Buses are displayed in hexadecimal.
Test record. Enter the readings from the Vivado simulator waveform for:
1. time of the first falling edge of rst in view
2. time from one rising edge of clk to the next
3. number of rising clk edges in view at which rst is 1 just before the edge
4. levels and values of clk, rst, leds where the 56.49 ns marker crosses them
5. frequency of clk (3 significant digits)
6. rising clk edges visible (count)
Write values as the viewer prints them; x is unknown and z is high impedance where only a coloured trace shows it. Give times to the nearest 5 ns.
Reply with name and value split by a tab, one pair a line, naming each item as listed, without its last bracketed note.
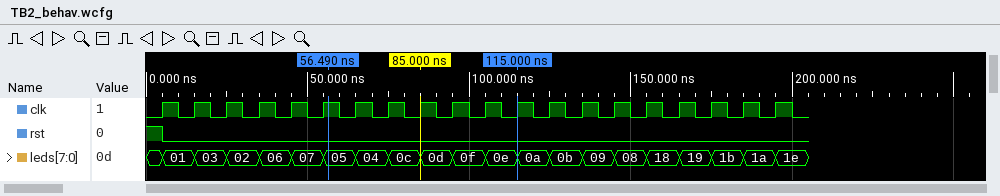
time of the first falling edge of rst in view	5 ns
time from one rising edge of clk to the next	10 ns
number of rising clk edges in view at which rst is 1 just before the edge	1
levels and values of clk, rst, leds where the 56.49 ns marker crosses them	clk=1, rst=0, leds=05
frequency of clk	100 MHz
rising clk edges visible	20
